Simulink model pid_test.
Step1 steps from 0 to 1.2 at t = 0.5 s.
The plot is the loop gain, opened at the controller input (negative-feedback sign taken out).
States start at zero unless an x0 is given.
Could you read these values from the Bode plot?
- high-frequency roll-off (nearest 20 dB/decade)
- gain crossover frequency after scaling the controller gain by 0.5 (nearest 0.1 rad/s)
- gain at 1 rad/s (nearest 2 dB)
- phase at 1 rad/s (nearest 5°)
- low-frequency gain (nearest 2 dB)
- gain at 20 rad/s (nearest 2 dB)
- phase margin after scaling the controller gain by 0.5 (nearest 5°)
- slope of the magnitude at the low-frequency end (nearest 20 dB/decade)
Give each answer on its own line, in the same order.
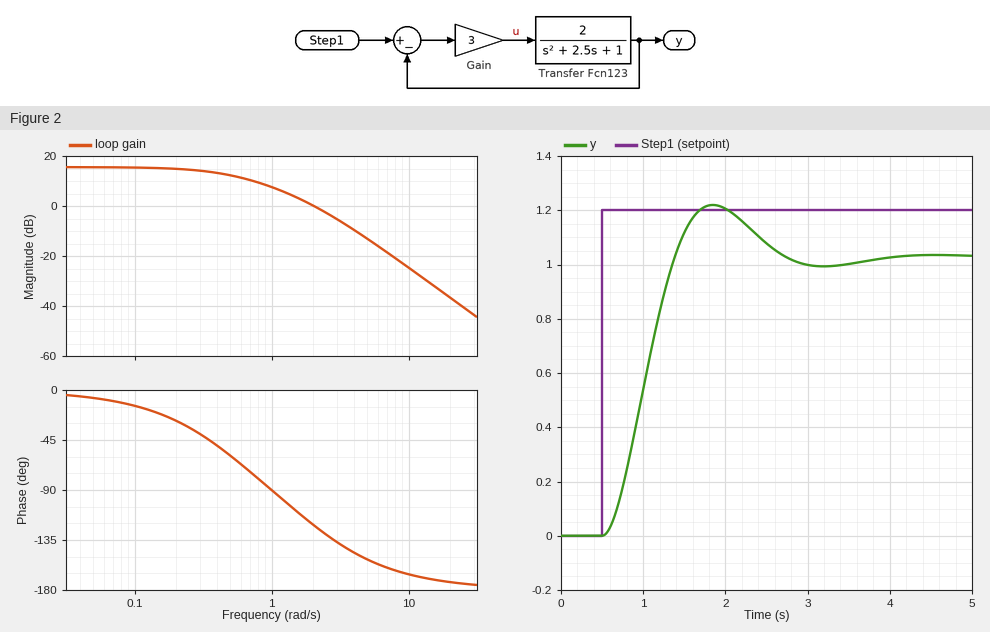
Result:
-40 dB/decade
1.2 rad/s
8 dB
-90°
16 dB
-36 dB
80°
0 dB/decade
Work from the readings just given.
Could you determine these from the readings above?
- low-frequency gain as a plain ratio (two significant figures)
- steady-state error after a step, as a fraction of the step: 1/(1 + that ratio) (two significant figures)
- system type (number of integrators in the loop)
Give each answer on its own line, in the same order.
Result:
6.3
0.14
0
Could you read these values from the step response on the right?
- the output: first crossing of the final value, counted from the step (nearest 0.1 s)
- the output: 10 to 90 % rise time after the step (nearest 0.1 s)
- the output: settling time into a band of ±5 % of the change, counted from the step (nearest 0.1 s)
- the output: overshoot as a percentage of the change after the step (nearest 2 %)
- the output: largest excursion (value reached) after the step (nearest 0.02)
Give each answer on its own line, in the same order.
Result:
0.9 s
0.6 s
2.0 s
18 %
1.22
